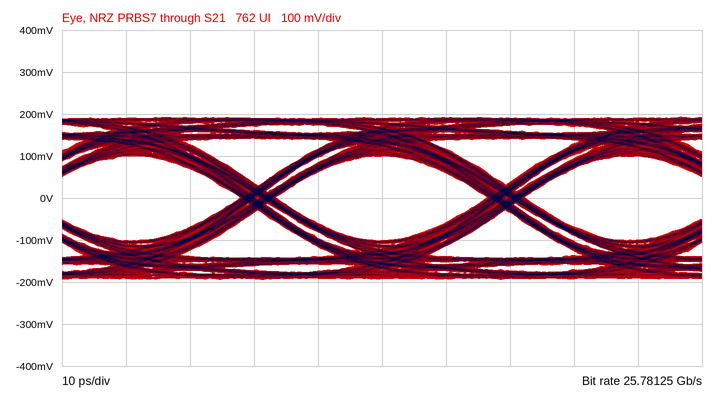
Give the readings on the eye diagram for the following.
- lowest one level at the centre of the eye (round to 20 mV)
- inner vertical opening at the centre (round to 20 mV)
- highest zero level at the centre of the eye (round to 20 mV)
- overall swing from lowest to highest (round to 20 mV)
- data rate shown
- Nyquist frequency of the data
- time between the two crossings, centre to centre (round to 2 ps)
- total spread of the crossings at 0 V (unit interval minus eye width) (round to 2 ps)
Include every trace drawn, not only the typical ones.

100 mV
200 mV
-100 mV
380 mV
25.78125 Gb/s
12.89062 GHz
38 ps
6 ps
